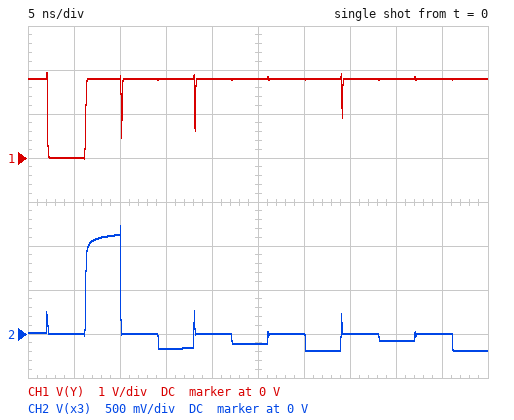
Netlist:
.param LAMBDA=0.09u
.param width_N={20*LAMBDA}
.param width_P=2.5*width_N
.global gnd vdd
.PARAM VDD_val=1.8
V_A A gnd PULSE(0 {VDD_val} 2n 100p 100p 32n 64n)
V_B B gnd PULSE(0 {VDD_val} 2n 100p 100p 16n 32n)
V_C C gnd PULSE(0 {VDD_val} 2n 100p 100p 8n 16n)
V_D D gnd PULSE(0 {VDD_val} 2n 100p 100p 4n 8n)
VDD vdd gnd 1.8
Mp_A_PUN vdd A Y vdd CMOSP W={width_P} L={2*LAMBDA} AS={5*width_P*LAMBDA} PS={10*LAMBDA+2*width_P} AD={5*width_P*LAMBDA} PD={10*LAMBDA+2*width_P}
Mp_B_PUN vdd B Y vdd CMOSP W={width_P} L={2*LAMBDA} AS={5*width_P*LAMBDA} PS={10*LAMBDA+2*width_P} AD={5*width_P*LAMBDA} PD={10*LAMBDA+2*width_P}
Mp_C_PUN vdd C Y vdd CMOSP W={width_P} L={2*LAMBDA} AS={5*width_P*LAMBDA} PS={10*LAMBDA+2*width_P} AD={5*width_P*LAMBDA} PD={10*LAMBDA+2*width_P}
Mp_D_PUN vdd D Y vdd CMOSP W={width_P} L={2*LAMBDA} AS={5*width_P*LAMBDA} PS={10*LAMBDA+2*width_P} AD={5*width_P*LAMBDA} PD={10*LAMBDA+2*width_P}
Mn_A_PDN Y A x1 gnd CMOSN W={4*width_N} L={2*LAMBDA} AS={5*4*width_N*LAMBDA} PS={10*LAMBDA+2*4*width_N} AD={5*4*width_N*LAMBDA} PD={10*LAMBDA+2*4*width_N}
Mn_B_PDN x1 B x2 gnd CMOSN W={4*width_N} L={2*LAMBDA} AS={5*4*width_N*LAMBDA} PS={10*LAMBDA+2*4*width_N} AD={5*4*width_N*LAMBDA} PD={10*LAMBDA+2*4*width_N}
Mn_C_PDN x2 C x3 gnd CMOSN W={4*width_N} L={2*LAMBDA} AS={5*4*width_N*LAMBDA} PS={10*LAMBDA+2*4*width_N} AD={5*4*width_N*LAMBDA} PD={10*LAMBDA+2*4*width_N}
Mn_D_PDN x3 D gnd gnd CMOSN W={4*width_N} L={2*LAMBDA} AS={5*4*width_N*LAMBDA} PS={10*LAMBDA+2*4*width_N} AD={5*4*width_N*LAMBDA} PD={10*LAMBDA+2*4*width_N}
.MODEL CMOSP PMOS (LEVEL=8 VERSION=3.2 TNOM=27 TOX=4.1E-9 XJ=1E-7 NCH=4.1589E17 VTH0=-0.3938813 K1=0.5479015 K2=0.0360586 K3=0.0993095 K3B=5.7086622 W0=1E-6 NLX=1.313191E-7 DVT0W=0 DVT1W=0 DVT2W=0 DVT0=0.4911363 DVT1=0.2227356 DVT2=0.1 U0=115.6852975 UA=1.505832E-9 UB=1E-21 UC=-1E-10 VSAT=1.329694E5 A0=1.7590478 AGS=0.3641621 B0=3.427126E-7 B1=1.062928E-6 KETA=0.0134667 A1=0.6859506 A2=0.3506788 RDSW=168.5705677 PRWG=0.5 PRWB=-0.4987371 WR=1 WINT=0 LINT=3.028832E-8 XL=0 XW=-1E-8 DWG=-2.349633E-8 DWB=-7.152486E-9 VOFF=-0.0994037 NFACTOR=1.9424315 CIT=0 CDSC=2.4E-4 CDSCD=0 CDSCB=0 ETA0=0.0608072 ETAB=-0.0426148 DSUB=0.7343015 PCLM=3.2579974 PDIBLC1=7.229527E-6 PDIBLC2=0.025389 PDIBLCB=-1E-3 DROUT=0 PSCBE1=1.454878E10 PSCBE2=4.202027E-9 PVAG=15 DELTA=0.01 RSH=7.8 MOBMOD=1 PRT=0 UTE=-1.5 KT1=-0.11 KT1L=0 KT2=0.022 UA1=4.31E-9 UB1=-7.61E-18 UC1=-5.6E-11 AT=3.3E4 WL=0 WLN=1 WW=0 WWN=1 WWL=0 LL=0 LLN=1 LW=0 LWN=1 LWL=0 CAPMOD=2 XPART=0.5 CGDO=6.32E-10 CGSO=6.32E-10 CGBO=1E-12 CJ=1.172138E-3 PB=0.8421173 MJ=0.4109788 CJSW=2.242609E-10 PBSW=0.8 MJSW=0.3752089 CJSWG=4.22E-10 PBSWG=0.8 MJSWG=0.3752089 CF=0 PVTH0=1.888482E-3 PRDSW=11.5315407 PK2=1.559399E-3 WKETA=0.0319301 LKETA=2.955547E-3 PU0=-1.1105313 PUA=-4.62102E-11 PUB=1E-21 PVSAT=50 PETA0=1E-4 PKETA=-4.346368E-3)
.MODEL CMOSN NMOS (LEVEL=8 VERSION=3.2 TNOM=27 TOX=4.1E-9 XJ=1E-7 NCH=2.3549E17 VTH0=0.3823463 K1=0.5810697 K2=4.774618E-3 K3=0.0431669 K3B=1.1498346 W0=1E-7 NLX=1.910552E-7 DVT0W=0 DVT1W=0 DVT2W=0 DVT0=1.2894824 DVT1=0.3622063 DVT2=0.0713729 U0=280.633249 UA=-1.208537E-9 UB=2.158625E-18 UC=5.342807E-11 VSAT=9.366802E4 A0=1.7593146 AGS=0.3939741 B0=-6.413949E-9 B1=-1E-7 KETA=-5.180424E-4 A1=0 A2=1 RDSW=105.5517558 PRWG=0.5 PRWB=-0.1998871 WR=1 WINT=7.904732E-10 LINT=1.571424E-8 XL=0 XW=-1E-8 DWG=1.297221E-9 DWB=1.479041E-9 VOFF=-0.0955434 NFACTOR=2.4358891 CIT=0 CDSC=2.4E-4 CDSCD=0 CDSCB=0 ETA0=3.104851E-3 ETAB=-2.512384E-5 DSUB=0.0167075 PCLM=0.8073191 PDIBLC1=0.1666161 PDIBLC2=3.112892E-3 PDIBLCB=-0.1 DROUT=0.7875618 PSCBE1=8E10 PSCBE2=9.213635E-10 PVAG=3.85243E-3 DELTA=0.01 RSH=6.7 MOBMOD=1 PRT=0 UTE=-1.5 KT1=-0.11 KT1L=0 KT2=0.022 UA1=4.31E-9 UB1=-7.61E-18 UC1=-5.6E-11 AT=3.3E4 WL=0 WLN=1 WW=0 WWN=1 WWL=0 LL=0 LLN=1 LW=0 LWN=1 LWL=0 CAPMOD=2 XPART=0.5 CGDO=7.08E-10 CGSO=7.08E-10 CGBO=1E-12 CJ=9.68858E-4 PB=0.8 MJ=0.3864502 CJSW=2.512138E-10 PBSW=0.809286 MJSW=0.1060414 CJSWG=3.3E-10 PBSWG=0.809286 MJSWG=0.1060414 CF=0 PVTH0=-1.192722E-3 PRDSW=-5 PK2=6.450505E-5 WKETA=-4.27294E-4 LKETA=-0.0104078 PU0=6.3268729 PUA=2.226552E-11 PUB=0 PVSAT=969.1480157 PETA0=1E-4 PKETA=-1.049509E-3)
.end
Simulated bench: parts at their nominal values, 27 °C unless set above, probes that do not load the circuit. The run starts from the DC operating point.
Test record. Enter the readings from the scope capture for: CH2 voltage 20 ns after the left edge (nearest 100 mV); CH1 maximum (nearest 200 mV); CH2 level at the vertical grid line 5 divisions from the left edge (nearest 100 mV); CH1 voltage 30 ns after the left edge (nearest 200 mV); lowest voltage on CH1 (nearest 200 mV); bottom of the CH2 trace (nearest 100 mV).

0 V
2.0 V
-100 mV
1.8 V
0 V
-200 mV
